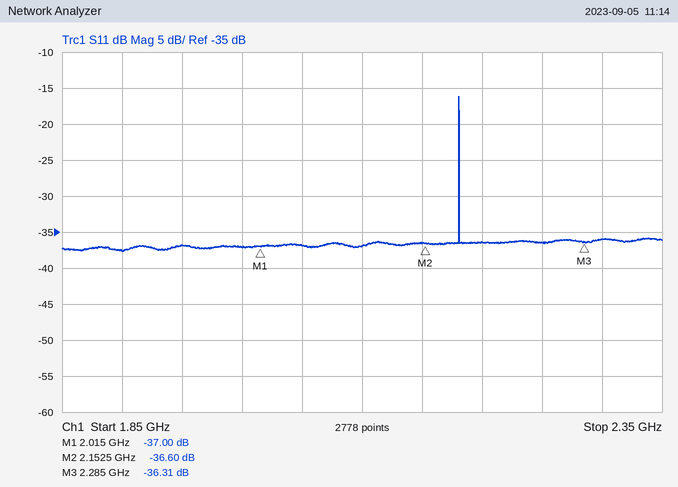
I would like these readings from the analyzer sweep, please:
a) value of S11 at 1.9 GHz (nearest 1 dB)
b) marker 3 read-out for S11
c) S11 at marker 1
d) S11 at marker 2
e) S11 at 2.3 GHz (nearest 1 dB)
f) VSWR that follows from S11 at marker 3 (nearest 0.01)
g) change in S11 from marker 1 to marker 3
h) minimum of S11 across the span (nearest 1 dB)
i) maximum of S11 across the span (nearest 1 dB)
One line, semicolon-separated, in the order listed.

-38 dB; -36.31 dB; -37.00 dB; -36.60 dB; -36 dB; 1.03; 0.69 dB; -38 dB; -16 dB
